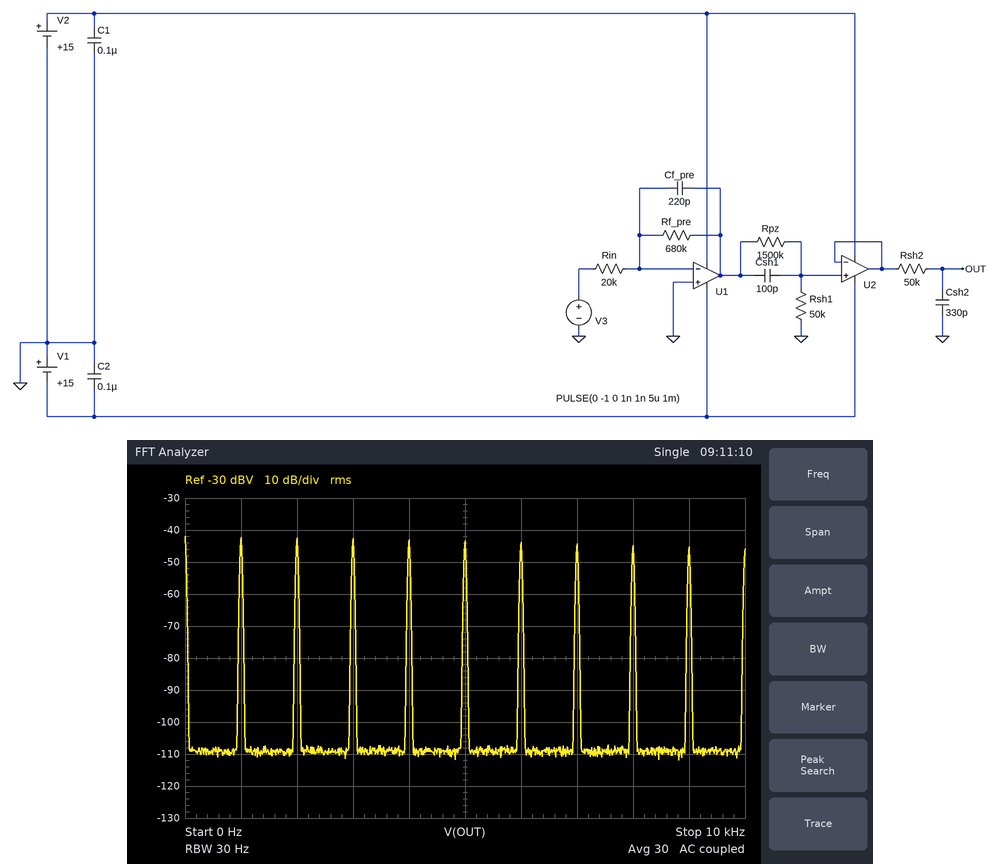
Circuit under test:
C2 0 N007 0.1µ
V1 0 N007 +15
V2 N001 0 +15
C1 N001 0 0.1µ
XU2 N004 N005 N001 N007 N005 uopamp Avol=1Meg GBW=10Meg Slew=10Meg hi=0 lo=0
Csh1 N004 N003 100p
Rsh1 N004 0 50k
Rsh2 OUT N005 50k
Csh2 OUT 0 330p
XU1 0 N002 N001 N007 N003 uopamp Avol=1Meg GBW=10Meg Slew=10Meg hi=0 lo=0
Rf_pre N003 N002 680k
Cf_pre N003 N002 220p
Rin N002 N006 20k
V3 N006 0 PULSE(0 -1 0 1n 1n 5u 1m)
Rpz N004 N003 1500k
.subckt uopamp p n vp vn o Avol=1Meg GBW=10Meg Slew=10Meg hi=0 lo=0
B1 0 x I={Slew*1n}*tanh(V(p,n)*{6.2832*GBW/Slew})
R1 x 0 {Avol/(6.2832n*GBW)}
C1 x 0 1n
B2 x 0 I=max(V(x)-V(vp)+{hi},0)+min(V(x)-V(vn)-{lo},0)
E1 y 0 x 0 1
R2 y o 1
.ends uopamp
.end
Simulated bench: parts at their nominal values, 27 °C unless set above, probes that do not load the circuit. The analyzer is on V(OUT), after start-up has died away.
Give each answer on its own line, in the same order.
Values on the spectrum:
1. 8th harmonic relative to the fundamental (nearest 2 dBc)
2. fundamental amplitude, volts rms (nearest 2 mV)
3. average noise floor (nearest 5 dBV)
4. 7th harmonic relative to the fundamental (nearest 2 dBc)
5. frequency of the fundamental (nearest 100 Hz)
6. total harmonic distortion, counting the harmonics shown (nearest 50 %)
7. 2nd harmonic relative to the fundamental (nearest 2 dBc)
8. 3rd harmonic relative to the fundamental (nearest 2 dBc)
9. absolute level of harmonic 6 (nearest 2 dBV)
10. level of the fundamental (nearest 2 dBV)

-2 dBc
8 mV
-110 dBV
-2 dBc
1.0 kHz
250 %
0 dBc
0 dBc
-44 dBV
-42 dBV
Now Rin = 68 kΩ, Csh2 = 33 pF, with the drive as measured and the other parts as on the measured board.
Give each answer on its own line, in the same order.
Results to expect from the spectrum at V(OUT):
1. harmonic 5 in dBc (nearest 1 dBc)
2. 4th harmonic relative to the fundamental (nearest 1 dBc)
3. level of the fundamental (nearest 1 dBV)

0 dBc
0 dBc
-53 dBV
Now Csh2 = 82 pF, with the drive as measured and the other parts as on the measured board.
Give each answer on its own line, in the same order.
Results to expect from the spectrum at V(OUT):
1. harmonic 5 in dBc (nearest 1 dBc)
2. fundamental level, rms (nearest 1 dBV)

0 dBc
-42 dBV
